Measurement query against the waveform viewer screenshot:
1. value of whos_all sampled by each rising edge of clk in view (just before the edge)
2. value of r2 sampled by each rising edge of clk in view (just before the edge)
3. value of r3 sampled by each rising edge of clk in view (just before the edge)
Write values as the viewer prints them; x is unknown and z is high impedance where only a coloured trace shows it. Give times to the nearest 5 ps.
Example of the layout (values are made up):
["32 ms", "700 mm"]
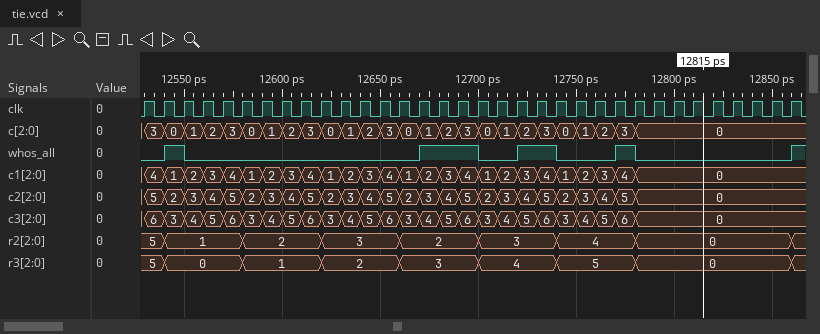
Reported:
["0 0 1 0 0 0 0 0 0 0 0 0 0 0 0 1 1 1 0 0 1 1 0 0 0 1 0 0 0 0 0 0 0 0", "5, 5, 1, 1, 1, 1, 2, 2, 2, 2, 3, 3, 3, 3, 2, 2, 2, 2, 3, 3, 3, 3, 4, 4, 4, 4, 0, 0, 0, 0, 0, 0, 0, 0", "5, 5, 0, 0, 0, 0, 1, 1, 1, 1, 2, 2, 2, 2, 3, 3, 3, 3, 4, 4, 4, 4, 5, 5, 5, 5, 0, 0, 0, 0, 0, 0, 0, 0"]
